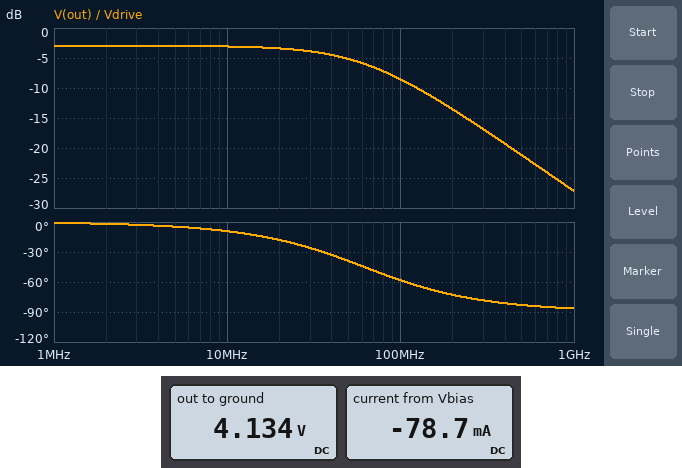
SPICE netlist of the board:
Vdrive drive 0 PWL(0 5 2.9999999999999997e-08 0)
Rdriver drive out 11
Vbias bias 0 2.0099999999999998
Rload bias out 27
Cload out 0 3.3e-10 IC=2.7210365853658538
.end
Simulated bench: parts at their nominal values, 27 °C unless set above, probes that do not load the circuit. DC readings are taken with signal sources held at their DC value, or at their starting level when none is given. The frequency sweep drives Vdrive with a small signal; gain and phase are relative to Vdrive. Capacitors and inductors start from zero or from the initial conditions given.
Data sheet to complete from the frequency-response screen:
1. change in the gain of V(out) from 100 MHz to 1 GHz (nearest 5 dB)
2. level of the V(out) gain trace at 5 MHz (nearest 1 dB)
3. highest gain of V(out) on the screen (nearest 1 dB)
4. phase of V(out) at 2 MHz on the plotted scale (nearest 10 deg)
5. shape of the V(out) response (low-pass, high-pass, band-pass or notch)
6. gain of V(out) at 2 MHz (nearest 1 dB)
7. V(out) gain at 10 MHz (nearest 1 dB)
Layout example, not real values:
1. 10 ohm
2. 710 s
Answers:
1. -20 dB
2. -3 dB
3. -3 dB
4. 0 deg
5. low-pass
6. -3 dB
7. -3 dB
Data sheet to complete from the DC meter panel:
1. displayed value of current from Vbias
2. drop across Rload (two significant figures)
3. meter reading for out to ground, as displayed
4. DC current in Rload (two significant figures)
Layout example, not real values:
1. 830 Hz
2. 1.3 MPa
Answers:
1. -78.7 mA
2. 2.1 V
3. 4.134 V
4. 79 mA
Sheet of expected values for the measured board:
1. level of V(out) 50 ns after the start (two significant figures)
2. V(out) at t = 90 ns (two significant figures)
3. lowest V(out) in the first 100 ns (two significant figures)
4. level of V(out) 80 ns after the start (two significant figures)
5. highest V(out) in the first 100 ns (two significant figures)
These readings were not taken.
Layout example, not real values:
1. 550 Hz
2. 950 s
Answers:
1. 580 mV
2. 580 mV
3. 580 mV
4. 580 mV
5. 3.6 V
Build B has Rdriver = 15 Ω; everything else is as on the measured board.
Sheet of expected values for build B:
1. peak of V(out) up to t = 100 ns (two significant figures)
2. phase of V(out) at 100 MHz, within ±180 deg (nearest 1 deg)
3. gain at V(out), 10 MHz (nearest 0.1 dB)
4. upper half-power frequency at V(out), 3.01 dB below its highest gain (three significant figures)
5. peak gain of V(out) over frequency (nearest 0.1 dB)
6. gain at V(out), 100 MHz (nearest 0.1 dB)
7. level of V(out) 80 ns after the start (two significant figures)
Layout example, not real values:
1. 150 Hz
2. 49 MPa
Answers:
1. 3.4 V
2. -63 deg
3. -4.0 dB
4. 50.0 MHz
5. -3.8 dB
6. -10.8 dB
7. 720 mV
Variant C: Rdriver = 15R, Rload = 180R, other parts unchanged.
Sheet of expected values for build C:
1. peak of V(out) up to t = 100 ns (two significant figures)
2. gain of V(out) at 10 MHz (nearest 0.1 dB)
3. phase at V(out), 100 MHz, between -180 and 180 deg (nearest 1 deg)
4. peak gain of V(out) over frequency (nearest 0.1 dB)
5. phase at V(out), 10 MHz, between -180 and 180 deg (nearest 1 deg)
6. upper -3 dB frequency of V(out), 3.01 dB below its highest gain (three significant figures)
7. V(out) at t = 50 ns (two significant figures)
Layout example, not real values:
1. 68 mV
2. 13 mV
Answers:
1. 3.8 V
2. -1.0 dB
3. -71 deg
4. -0.7 dB
5. -16 deg
6. 34.8 MHz
7. 160 mV
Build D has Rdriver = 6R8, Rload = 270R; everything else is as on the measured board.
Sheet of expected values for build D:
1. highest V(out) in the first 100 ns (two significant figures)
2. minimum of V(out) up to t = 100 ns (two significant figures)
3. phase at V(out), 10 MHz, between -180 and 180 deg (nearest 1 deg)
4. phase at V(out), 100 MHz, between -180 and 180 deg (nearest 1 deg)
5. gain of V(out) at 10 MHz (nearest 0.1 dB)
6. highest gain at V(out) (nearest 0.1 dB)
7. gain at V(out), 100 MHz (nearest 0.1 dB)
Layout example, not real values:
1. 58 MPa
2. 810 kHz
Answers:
1. 4.2 V
2. 49 mV
3. -8 deg
4. -54 deg
5. -0.3 dB
6. -0.2 dB
7. -4.8 dB
